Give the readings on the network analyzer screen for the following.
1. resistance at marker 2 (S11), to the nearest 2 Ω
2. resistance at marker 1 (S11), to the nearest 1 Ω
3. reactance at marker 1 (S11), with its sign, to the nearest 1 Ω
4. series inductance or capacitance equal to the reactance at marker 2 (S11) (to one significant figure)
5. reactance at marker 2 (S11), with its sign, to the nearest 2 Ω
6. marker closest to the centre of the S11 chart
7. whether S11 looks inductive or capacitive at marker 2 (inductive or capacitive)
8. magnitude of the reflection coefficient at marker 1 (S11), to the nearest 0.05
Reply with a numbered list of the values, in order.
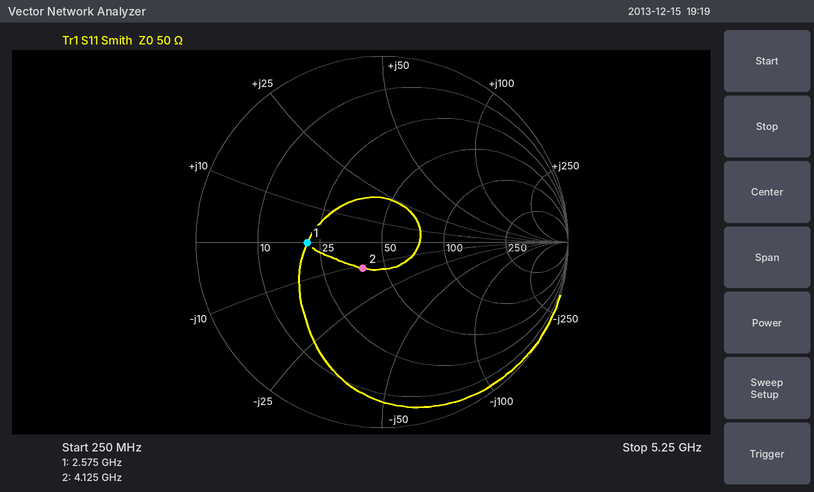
1. 40 Ω
2. 21 Ω
3. 0 Ω
4. 3 pF
5. -12 Ω
6. marker 2
7. capacitive
8. 0.40
